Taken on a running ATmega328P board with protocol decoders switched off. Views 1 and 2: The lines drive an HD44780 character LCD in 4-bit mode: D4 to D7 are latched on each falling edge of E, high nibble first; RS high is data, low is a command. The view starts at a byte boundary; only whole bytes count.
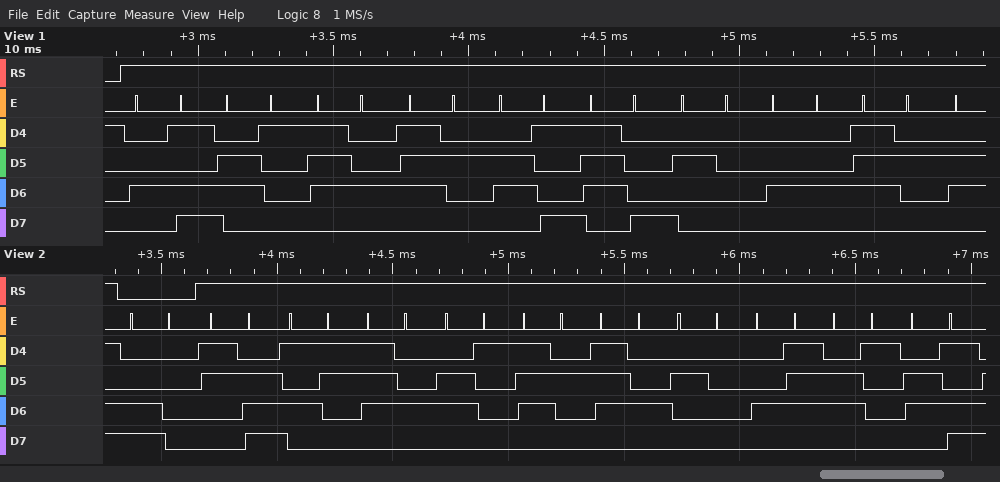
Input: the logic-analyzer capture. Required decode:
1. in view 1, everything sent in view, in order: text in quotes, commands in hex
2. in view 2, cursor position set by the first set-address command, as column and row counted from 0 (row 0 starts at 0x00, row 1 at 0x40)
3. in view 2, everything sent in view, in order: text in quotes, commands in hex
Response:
"Matrix Dr"
column 0, row 1
0xC0 ">Start Gam"
